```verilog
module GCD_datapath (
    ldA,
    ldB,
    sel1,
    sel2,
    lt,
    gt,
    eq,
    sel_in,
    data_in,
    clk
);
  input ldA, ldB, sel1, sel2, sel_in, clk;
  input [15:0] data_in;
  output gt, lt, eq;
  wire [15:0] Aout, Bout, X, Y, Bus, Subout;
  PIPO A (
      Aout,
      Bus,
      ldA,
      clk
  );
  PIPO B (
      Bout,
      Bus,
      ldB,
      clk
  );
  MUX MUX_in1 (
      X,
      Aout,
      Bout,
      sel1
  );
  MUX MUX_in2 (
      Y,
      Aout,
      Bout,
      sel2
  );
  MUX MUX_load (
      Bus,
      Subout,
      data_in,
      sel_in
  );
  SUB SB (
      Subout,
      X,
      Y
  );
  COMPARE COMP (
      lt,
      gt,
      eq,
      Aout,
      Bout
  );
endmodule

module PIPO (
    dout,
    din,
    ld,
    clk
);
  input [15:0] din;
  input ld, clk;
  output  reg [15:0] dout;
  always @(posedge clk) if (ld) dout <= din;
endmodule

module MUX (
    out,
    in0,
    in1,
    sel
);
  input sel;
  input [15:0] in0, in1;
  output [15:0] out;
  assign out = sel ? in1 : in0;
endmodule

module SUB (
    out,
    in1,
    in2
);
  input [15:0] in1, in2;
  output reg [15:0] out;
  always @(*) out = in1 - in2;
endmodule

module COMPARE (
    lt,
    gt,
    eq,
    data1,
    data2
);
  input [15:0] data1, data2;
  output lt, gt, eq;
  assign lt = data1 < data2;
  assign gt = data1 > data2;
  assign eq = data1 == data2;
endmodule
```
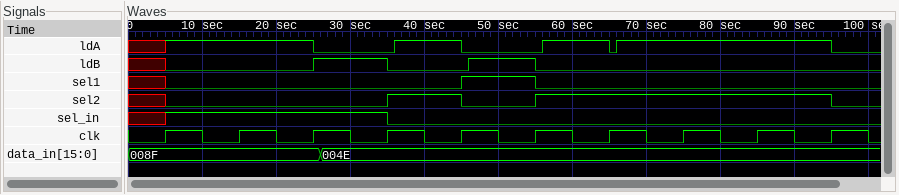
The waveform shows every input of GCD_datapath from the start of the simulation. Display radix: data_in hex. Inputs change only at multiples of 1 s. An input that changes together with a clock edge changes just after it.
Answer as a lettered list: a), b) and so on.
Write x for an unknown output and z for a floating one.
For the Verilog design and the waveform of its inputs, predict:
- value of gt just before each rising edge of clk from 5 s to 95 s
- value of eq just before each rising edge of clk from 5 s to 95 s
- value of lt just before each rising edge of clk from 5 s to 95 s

a) x x x x 1 0 1 1 1 1
b) x x x x 0 0 0 0 0 0
c) x x x x 0 1 0 0 0 0
